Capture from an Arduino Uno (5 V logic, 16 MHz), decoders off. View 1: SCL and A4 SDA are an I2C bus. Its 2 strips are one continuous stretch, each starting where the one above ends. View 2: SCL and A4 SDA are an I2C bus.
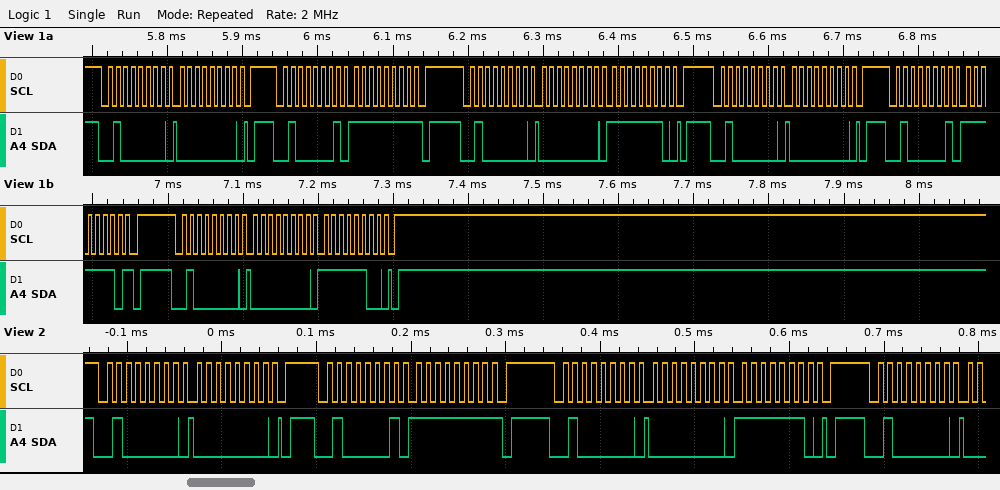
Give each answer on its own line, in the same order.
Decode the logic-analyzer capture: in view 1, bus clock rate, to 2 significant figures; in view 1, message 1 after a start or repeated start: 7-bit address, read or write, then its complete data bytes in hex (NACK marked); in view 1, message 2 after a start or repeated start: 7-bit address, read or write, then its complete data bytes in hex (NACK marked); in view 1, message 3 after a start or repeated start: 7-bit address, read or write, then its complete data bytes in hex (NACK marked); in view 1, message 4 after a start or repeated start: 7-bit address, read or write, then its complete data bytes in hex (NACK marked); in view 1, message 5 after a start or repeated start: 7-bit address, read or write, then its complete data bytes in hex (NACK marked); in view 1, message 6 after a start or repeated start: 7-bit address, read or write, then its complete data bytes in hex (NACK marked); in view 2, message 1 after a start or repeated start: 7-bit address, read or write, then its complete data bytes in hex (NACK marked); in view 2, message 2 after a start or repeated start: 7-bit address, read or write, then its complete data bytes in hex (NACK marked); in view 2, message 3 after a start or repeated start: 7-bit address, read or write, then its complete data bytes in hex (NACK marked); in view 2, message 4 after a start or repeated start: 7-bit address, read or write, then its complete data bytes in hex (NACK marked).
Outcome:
100 kHz
0x20 write: 00
0x20 read: FF NACK
0x20 write: 00 FE
0x20 write: 00
0x20 read: FE NACK
0x20 write: 00 FC
0x20 write: 00
0x20 read: FF NACK
0x20 write: 00 FE
0x20 write
